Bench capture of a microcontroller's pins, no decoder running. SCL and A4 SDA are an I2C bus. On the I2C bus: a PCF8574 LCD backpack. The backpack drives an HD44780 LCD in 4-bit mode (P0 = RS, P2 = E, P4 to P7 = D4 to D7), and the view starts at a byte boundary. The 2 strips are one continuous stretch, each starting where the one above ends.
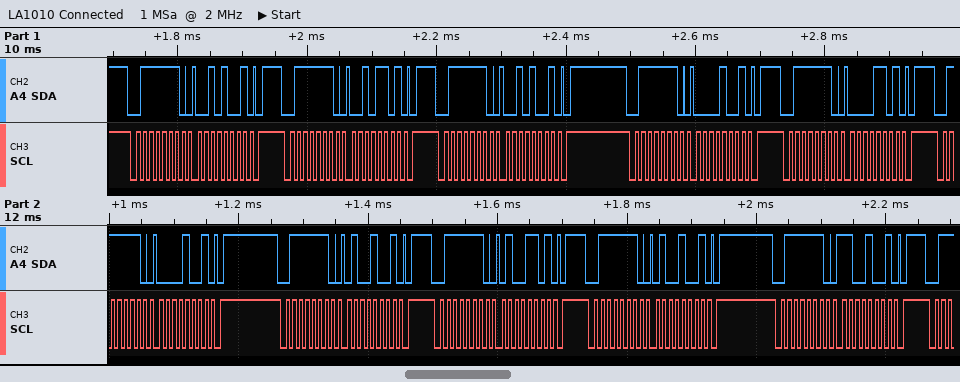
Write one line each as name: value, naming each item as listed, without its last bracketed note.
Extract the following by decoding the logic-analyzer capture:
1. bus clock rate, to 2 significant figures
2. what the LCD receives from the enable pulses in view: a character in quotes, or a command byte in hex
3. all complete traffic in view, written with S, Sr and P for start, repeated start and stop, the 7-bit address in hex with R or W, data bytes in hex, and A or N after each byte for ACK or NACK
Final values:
bus clock rate, to 2 significant figures: 100 kHz
what the LCD receives from the enable pulses in view: a character in quotes, or a command byte in hex: ' '
all complete traffic in view, written with S, Sr and P for start, repeated start and stop, the 7-bit address in hex with R or W, data bytes in hex, and A or N after each byte for ACK or NACK: S 3FW A 29 A P S 3FW A 2D A P S 3FW A 29 A P S 3FW A 09 A P S 3FW A 0D A P S 3FW A 09 A P S 3FW A 49 A P S 3FW A 4D A P S 3FW A 49 A P S 3FW A C9 A P
